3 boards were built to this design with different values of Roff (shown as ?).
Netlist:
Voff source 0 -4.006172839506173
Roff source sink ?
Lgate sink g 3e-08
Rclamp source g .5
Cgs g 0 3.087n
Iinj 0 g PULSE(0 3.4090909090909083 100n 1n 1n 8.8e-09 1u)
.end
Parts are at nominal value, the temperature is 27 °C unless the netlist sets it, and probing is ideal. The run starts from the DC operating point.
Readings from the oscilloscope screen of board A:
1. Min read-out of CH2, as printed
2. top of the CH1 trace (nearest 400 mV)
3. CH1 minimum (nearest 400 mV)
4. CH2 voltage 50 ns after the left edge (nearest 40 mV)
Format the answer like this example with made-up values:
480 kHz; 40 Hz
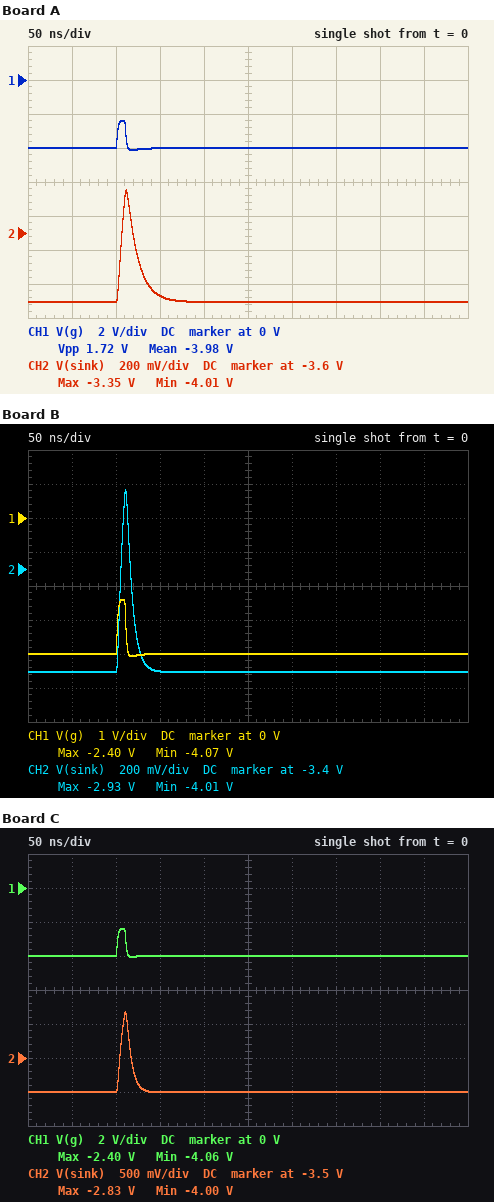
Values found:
-4.01 V; -2.4 V; -4.0 V; -4.00 V
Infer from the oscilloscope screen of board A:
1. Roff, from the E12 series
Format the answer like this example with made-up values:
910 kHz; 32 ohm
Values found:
1.8 Ω
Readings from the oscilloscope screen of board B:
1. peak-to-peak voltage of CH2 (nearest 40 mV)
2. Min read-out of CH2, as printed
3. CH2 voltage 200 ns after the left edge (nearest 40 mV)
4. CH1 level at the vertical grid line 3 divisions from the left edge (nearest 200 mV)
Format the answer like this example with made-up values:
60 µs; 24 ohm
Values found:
1.08 V; -4.01 V; -4.00 V; -4.0 V
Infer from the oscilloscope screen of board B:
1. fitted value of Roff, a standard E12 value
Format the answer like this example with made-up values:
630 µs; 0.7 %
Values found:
3.9 Ω
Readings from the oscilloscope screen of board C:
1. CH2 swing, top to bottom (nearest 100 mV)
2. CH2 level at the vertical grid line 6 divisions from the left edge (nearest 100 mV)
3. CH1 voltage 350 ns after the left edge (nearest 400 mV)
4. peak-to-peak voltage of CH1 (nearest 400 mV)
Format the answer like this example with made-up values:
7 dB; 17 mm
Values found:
1.2 V; -4.0 V; -4.0 V; 1.6 V
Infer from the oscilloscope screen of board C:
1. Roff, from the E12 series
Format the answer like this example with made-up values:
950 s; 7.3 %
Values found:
4.7 Ω
